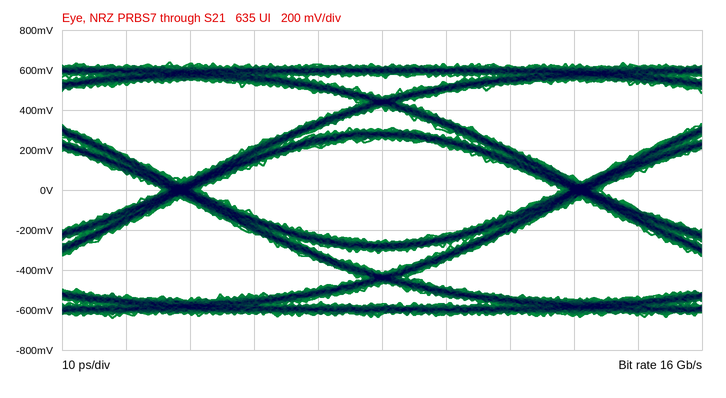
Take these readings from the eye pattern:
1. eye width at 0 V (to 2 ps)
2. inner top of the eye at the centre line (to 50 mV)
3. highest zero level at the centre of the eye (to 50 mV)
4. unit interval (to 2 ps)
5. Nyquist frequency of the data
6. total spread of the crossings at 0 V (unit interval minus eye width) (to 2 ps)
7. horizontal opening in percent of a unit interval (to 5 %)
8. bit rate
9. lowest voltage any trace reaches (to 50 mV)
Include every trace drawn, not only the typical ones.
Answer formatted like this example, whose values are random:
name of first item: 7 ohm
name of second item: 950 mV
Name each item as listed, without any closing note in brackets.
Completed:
eye width at 0 V: 56 ps
inner top of the eye at the centre line: 250 mV
highest zero level at the centre of the eye: -250 mV
unit interval: 62 ps
Nyquist frequency of the data: 8 GHz
total spread of the crossings at 0 V (unit interval minus eye width): 6 ps
horizontal opening in percent of a unit interval: 90 %
bit rate: 16 Gb/s
lowest voltage any trace reaches: -650 mV
